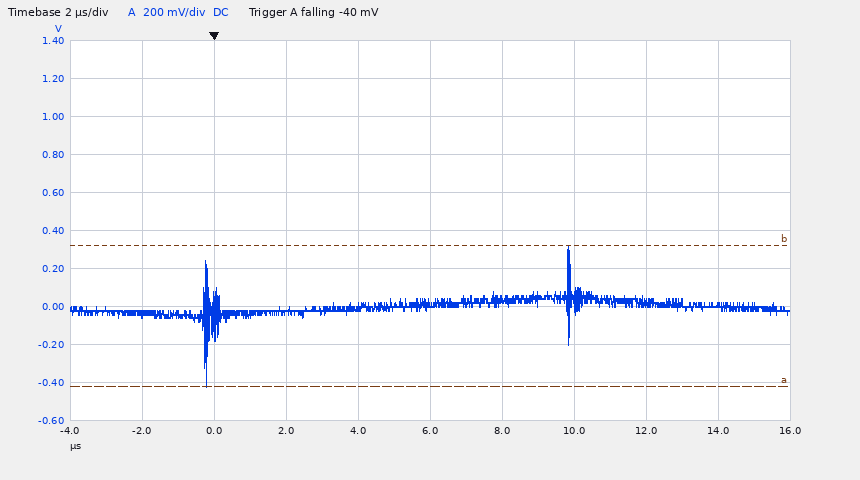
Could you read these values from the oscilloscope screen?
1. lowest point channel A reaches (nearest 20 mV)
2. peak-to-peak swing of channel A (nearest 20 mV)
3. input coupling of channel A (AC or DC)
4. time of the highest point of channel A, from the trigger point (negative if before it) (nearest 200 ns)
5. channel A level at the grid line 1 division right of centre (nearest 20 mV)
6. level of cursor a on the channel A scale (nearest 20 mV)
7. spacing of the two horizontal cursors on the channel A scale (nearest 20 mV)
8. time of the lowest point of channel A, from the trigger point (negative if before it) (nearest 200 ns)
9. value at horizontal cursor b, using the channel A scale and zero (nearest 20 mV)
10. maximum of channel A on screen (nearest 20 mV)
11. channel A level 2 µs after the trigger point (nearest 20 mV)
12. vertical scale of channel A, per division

-420 mV
740 mV
DC
+9.8 µs
40 mV
-420 mV
740 mV
-200 ns
320 mV
320 mV
-20 mV
200 mV
